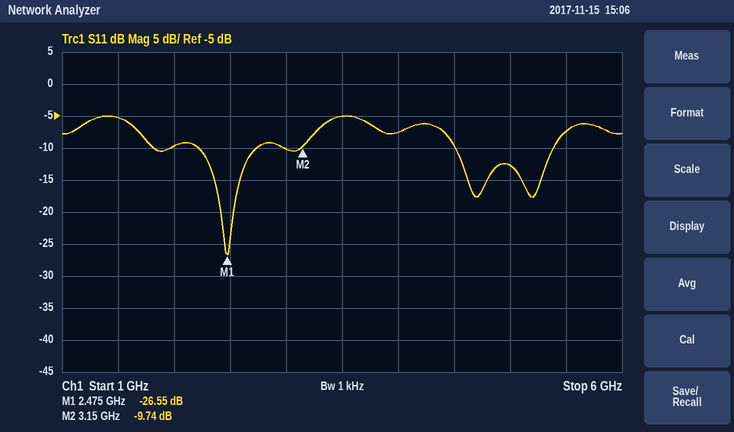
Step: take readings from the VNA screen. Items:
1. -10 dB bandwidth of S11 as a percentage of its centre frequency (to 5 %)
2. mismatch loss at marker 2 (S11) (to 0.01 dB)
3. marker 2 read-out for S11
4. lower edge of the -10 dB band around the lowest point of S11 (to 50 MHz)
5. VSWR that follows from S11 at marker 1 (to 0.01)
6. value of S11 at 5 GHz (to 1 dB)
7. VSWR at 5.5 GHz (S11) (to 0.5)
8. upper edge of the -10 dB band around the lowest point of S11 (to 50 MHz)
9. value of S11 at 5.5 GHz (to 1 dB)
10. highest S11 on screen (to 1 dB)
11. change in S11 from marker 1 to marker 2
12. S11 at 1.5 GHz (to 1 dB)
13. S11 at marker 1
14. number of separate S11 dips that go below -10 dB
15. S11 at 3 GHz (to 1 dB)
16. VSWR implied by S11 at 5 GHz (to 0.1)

20 %
0.49 dB
-9.74 dB
2.20 GHz
1.10
-13 dB
2.5
2.75 GHz
-7 dB
-5 dB
16.81 dB
-5 dB
-26.55 dB
3
-10 dB
1.6
